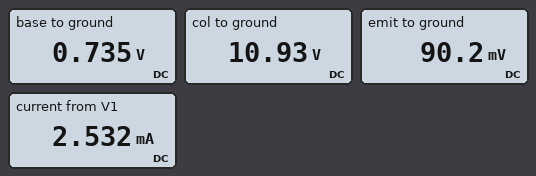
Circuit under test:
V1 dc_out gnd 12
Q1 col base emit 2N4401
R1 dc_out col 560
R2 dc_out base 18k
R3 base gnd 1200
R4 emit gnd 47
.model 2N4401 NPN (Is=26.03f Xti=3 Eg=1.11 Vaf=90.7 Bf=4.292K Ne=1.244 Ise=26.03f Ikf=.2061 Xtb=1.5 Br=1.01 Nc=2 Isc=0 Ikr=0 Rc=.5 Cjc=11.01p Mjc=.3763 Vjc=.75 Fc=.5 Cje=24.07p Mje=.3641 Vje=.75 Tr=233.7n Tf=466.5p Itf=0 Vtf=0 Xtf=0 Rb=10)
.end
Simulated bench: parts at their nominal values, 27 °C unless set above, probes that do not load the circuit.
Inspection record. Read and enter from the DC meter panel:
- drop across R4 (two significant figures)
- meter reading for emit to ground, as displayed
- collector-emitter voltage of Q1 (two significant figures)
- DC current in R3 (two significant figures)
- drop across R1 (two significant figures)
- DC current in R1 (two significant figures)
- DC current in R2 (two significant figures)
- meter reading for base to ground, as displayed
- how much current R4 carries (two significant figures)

90 mV
90.2 mV
11 V
610 µA
1.1 V
1.9 mA
630 µA
0.735 V
1.9 mA
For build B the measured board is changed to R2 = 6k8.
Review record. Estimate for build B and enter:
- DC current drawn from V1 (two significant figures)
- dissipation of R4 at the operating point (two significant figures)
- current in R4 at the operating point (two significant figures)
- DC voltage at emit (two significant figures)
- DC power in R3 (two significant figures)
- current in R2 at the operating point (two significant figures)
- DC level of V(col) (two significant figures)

21 mA
18 mW
20 mA
920 mV
2.2 mW
1.5 mA
1.1 V
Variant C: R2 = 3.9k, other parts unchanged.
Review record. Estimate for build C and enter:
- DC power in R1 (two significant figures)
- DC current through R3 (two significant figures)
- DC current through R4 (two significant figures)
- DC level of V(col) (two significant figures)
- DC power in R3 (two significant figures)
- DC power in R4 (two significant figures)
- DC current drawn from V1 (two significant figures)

210 mW
1.4 mA
21 mA
1.1 V
2.4 mW
20 mW
22 mA
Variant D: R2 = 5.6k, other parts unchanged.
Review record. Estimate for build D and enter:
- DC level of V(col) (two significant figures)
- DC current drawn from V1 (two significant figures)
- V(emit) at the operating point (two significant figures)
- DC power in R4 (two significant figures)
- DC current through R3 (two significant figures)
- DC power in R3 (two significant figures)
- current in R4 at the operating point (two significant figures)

1.1 V
21 mA
940 mV
19 mW
1.4 mA
2.3 mW
20 mA
